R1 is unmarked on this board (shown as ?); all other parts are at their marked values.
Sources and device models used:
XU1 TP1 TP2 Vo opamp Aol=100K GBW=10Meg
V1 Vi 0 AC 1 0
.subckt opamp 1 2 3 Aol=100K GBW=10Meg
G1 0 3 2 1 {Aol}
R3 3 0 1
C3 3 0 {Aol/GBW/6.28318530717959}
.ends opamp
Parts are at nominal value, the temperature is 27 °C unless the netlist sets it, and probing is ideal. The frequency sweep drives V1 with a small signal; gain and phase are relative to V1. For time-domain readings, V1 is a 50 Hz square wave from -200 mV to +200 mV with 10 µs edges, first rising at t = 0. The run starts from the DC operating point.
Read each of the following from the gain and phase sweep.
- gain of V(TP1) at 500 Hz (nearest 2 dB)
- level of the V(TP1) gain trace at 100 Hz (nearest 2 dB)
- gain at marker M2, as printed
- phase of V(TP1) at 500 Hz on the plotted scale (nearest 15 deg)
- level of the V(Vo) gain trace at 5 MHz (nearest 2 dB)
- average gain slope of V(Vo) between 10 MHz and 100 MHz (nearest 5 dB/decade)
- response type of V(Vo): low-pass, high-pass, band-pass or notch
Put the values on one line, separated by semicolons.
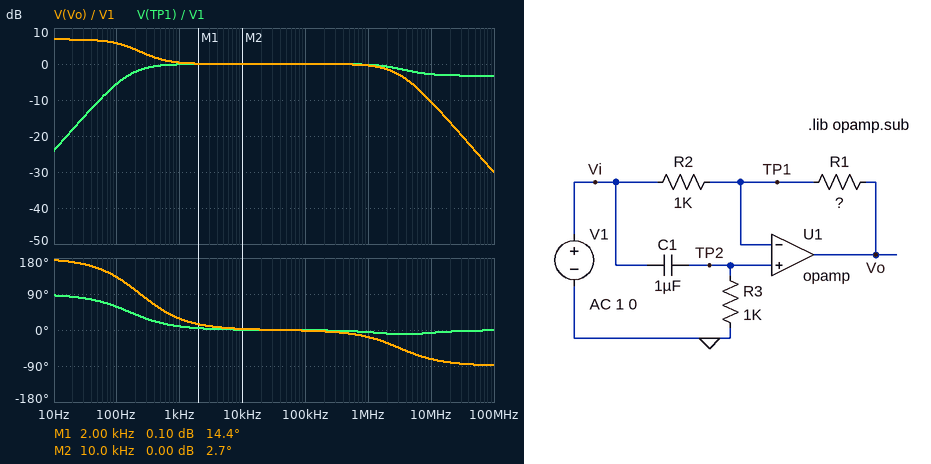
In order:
0 dB; -6 dB; 0.00 dB; 15 deg; -6 dB; -20 dB/decade; low-pass
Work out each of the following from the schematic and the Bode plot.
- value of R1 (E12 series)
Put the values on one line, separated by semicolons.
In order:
2.2 kΩ
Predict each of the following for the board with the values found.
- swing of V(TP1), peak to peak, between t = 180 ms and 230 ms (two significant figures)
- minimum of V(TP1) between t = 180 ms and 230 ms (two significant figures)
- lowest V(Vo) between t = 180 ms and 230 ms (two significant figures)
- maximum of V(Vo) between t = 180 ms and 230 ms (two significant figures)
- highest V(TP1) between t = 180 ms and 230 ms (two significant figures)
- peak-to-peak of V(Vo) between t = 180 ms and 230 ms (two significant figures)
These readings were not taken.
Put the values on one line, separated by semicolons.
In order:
800 mV; -400 mV; -830 mV; 830 mV; 400 mV; 1.7 V
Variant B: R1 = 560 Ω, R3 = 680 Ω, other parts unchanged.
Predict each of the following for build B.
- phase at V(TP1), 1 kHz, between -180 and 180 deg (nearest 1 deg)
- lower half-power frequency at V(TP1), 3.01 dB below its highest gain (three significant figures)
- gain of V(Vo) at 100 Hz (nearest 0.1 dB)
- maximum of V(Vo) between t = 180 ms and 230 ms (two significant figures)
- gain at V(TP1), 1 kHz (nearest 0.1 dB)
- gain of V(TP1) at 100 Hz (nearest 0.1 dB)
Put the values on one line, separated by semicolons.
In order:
13 deg; 234 Hz; -3.8 dB; 510 mV; -0.2 dB; -8.1 dB
